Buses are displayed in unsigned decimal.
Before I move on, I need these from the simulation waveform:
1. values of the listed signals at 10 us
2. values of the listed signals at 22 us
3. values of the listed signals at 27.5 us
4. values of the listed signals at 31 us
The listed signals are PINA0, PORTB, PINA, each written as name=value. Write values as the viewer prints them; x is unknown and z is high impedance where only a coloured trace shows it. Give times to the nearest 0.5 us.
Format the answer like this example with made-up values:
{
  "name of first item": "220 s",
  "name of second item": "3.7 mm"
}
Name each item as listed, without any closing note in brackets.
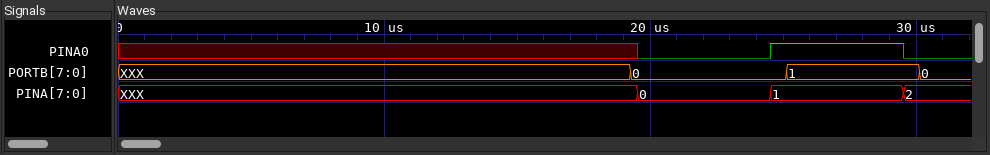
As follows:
{
  "values of the listed signals at 10 us": "PINA0=x, PORTB=XXX, PINA=XXX",
  "values of the listed signals at 22 us": "PINA0=0, PORTB=0, PINA=0",
  "values of the listed signals at 27.5 us": "PINA0=1, PORTB=1, PINA=1",
  "values of the listed signals at 31 us": "PINA0=0, PORTB=0, PINA=2"
}
